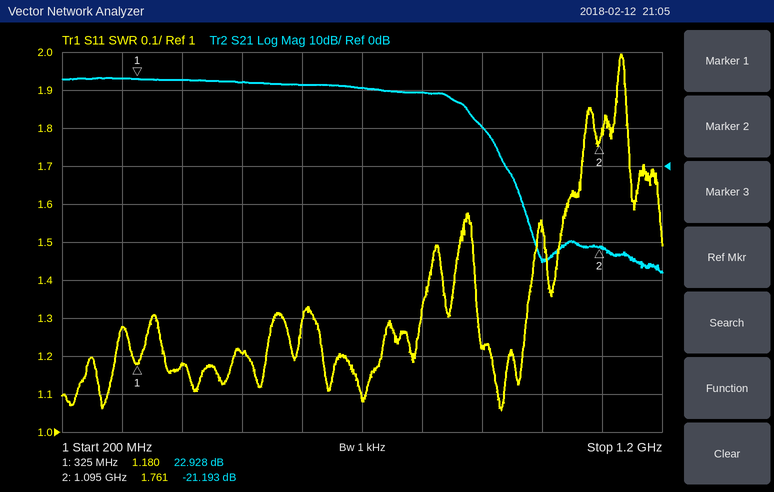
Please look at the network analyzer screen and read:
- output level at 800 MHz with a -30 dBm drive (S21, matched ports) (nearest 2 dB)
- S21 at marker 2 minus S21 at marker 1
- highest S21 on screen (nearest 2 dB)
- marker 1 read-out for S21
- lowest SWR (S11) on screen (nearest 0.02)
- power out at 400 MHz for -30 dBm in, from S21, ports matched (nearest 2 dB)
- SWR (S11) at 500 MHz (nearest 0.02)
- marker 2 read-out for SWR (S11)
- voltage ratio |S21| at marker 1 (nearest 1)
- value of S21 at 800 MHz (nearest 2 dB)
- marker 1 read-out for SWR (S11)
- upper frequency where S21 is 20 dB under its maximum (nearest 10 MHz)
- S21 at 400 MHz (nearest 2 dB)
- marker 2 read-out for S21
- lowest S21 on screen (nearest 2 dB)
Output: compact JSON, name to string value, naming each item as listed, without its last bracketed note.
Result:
{"output level at 800 MHz with a -30 dBm drive (S21, matched ports)": "-10 dBm", "S21 at marker 2 minus S21 at marker 1": "-44.121 dB", "highest S21 on screen": "24 dB", "marker 1 read-out for S21": "22.928 dB", "lowest SWR (S11) on screen": "1.06", "power out at 400 MHz for -30 dBm in, from S21, ports matched": "-8 dBm", "SWR (S11) at 500 MHz": "1.20", "marker 2 read-out for SWR": "1.761", "voltage ratio |S21| at marker 1": "14", "value of S21 at 800 MHz": "20 dB", "marker 1 read-out for SWR": "1.180", "upper frequency where S21 is 20 dB under its maximum": "930 MHz", "S21 at 400 MHz": "22 dB", "marker 2 read-out for S21": "-21.193 dB", "lowest S21 on screen": "-28 dB"}
